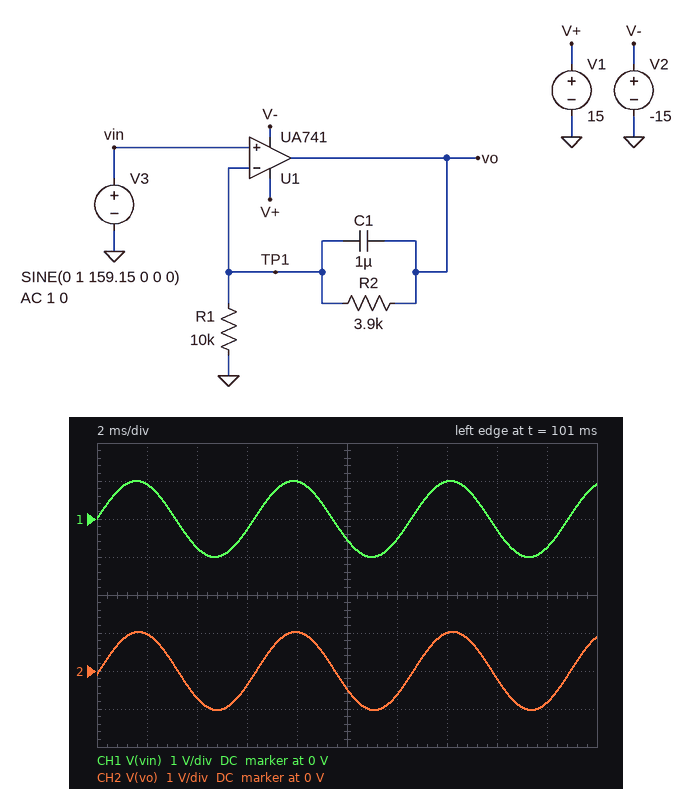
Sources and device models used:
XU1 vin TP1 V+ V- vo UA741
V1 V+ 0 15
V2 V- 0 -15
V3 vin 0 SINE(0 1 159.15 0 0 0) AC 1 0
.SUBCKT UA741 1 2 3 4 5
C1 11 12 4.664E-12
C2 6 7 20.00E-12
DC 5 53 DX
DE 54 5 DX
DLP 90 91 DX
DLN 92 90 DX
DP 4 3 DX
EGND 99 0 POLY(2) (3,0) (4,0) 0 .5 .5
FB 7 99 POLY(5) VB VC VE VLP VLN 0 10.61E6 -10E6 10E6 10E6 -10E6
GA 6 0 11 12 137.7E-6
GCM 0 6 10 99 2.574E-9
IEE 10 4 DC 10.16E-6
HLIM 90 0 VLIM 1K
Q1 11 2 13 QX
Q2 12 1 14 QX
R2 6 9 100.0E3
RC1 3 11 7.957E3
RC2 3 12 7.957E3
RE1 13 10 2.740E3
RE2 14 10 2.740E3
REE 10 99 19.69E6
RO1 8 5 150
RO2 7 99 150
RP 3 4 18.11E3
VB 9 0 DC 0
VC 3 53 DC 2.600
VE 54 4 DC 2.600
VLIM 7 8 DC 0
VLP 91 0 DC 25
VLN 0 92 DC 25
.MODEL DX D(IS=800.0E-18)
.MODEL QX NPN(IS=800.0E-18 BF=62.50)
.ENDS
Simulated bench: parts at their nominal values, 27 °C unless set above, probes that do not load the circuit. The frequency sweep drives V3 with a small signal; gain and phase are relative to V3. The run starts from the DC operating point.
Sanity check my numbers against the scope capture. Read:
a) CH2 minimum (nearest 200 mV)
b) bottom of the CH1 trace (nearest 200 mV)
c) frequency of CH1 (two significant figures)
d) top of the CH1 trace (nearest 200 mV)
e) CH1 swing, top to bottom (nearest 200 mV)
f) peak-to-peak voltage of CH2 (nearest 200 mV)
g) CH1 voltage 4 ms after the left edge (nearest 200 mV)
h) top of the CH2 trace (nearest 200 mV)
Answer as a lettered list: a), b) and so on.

a) -1.0 V
b) -1.0 V
c) 160 Hz
d) 1.0 V
e) 2.0 V
f) 2.0 V
g) -800 mV
h) 1.0 V
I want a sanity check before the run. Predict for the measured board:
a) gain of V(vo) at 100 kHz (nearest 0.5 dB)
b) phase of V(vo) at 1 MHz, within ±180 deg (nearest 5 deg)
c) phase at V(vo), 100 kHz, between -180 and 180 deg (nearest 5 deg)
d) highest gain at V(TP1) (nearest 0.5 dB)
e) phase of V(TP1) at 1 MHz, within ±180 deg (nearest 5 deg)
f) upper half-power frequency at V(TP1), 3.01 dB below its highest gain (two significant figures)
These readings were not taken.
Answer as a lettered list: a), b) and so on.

a) 0 dB
b) -60 deg
c) -5 deg
d) 0 dB
e) -60 deg
f) 1.5 MHz
